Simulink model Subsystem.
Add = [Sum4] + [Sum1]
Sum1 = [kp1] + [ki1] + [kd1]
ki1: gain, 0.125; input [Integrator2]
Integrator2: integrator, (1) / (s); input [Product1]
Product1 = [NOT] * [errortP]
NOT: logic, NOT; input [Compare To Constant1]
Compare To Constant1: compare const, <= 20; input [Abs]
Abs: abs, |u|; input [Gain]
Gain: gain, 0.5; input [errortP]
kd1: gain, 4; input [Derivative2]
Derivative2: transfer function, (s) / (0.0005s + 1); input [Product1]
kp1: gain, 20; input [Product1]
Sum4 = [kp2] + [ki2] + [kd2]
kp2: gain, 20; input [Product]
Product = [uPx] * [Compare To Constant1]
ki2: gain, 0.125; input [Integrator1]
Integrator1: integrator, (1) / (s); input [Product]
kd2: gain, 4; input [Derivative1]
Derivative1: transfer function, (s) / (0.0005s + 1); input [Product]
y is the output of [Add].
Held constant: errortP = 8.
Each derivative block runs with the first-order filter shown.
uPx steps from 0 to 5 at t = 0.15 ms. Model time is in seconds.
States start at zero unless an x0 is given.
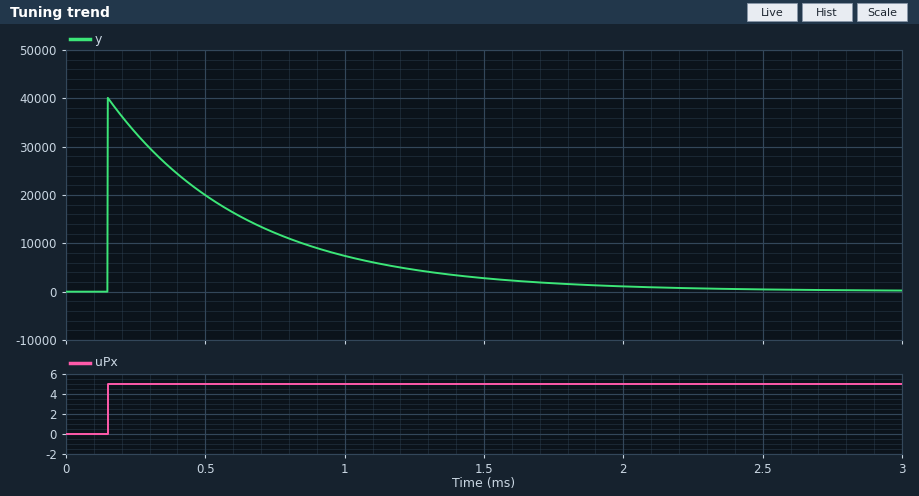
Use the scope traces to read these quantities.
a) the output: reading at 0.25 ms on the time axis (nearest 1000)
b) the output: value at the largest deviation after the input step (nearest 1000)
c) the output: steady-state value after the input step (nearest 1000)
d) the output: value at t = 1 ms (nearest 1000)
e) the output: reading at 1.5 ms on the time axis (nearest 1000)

33000
40000
0
7000
3000
